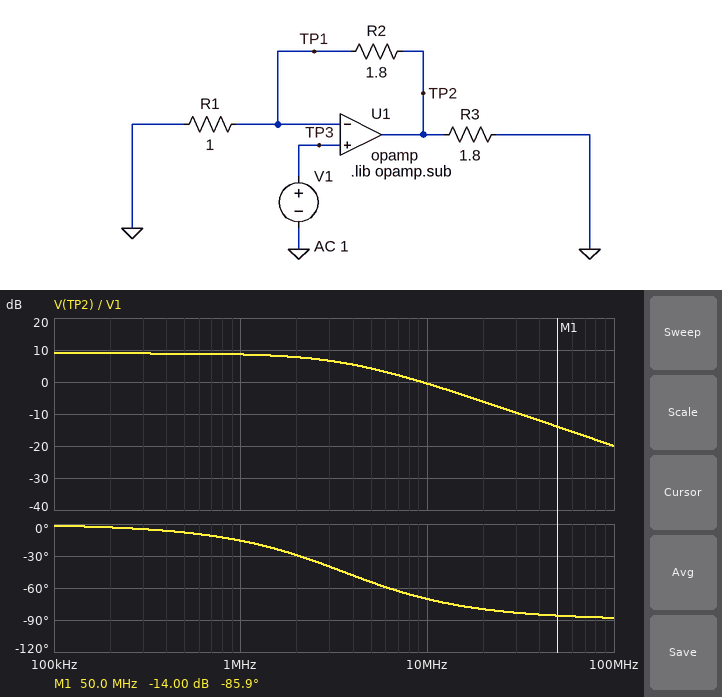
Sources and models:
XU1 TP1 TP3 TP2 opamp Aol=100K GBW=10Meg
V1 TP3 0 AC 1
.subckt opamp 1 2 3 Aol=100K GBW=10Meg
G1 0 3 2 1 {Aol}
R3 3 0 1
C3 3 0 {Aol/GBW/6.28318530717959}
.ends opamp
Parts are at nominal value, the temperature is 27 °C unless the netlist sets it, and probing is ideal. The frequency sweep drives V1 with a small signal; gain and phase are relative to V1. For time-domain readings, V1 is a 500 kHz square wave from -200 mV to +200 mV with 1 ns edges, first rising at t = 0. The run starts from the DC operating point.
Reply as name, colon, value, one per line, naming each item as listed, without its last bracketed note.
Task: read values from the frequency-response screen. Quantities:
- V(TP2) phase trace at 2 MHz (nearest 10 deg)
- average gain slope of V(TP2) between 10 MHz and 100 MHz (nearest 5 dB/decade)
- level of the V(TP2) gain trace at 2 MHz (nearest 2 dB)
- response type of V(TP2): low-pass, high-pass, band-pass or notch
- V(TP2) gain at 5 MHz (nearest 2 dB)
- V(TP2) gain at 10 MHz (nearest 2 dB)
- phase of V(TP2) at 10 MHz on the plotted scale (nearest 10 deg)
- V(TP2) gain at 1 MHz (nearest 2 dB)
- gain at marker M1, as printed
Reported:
V(TP2) phase trace at 2 MHz: -30 deg
average gain slope of V(TP2) between 10 MHz and 100 MHz: -20 dB/decade
level of the V(TP2) gain trace at 2 MHz: 8 dB
response type of V(TP2): low-pass, high-pass, band-pass or notch: low-pass
V(TP2) gain at 5 MHz: 4 dB
V(TP2) gain at 10 MHz: 0 dB
phase of V(TP2) at 10 MHz on the plotted scale: -70 deg
V(TP2) gain at 1 MHz: 8 dB
gain at marker M1, as printed: -14.00 dB
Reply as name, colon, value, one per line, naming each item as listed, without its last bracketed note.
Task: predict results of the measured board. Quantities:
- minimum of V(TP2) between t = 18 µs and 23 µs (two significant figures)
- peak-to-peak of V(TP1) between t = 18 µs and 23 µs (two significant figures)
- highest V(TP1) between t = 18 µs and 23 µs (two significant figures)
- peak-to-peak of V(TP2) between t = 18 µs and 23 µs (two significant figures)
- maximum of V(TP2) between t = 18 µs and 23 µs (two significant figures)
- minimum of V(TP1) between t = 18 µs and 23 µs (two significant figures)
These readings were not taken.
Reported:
minimum of V(TP2) between t = 18 µs and 23 µs: -560 mV
peak-to-peak of V(TP1) between t = 18 µs and 23 µs: 400 mV
highest V(TP1) between t = 18 µs and 23 µs: 200 mV
peak-to-peak of V(TP2) between t = 18 µs and 23 µs: 1.1 V
maximum of V(TP2) between t = 18 µs and 23 µs: 560 mV
minimum of V(TP1) between t = 18 µs and 23 µs: -200 mV
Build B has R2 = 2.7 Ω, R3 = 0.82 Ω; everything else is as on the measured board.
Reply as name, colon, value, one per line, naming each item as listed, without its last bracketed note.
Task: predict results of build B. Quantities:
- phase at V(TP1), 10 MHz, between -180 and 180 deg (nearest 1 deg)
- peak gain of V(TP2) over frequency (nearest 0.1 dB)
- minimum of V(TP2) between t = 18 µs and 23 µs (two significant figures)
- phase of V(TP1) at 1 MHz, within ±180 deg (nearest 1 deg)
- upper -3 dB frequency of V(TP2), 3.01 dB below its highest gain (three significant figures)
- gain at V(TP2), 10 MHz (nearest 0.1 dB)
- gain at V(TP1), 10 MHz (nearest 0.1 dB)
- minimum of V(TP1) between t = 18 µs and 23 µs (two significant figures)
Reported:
phase at V(TP1), 10 MHz, between -180 and 180 deg: -75 deg
peak gain of V(TP2) over frequency: 11.4 dB
minimum of V(TP2) between t = 18 µs and 23 µs: -740 mV
phase of V(TP1) at 1 MHz, within ±180 deg: -20 deg
upper -3 dB frequency of V(TP2), 3.01 dB below its highest gain: 2.70 MHz
gain at V(TP2), 10 MHz: -0.3 dB
gain at V(TP1), 10 MHz: -11.7 dB
minimum of V(TP1) between t = 18 µs and 23 µs: -200 mV
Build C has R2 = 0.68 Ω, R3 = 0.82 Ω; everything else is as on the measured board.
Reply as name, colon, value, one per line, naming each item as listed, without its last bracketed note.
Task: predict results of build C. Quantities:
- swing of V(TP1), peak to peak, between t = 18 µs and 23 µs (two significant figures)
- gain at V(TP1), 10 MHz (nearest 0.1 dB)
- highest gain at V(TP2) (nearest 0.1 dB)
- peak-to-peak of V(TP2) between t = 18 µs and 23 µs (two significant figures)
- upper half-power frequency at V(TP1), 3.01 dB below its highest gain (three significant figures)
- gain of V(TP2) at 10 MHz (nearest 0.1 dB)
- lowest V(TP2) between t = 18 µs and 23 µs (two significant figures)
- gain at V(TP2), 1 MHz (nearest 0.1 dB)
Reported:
swing of V(TP1), peak to peak, between t = 18 µs and 23 µs: 400 mV
gain at V(TP1), 10 MHz: -5.8 dB
highest gain at V(TP2): 4.5 dB
peak-to-peak of V(TP2) between t = 18 µs and 23 µs: 670 mV
upper half-power frequency at V(TP1), 3.01 dB below its highest gain: 5.95 MHz
gain of V(TP2) at 10 MHz: -1.3 dB
lowest V(TP2) between t = 18 µs and 23 µs: -340 mV
gain at V(TP2), 1 MHz: 4.4 dB
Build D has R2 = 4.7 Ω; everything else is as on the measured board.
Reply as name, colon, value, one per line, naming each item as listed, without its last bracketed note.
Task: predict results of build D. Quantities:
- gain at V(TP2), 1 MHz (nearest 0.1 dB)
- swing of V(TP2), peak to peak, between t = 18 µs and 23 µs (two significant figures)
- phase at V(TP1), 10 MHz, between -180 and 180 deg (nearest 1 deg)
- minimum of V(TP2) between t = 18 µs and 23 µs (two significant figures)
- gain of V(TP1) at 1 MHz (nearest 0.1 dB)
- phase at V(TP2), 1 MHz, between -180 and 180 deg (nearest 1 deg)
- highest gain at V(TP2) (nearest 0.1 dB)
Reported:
gain at V(TP2), 1 MHz: 13.9 dB
swing of V(TP2), peak to peak, between t = 18 µs and 23 µs: 2.3 V
phase at V(TP1), 10 MHz, between -180 and 180 deg: -80 deg
minimum of V(TP2) between t = 18 µs and 23 µs: -1.1 V
gain of V(TP1) at 1 MHz: -1.2 dB
phase at V(TP2), 1 MHz, between -180 and 180 deg: -30 deg
highest gain at V(TP2): 15.1 dB
